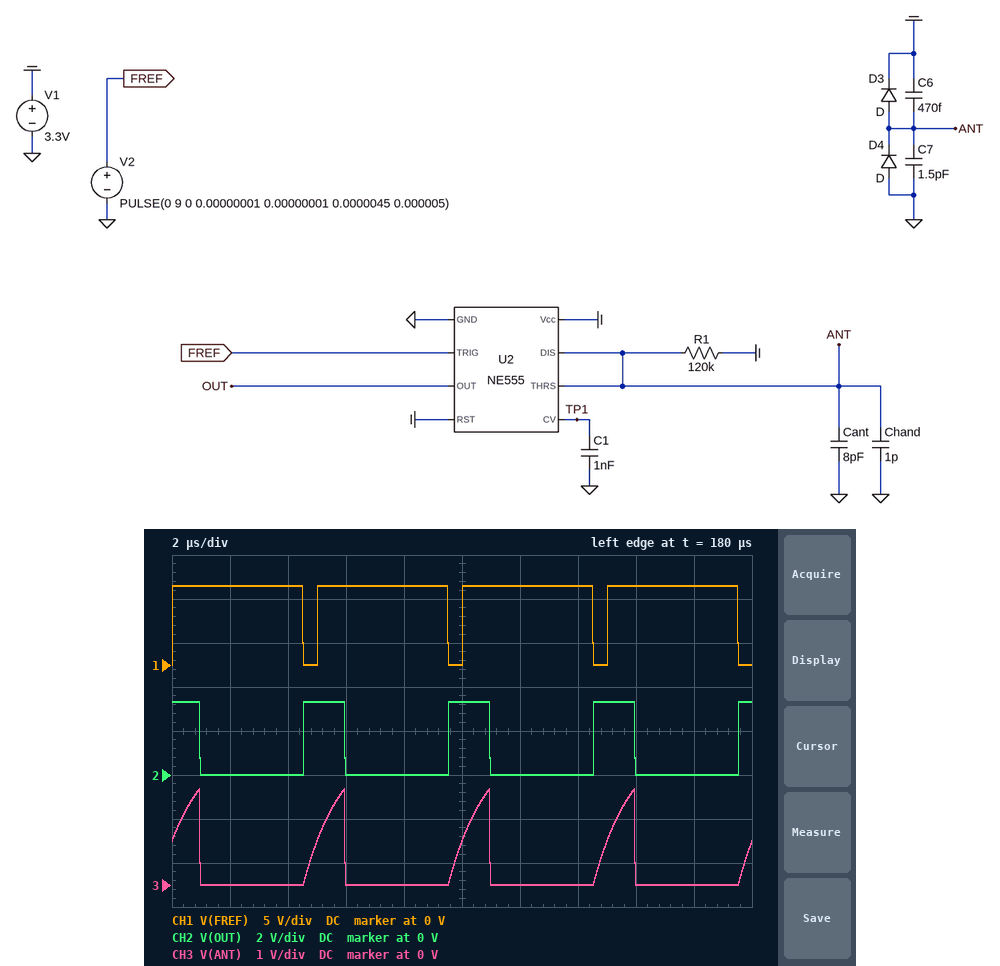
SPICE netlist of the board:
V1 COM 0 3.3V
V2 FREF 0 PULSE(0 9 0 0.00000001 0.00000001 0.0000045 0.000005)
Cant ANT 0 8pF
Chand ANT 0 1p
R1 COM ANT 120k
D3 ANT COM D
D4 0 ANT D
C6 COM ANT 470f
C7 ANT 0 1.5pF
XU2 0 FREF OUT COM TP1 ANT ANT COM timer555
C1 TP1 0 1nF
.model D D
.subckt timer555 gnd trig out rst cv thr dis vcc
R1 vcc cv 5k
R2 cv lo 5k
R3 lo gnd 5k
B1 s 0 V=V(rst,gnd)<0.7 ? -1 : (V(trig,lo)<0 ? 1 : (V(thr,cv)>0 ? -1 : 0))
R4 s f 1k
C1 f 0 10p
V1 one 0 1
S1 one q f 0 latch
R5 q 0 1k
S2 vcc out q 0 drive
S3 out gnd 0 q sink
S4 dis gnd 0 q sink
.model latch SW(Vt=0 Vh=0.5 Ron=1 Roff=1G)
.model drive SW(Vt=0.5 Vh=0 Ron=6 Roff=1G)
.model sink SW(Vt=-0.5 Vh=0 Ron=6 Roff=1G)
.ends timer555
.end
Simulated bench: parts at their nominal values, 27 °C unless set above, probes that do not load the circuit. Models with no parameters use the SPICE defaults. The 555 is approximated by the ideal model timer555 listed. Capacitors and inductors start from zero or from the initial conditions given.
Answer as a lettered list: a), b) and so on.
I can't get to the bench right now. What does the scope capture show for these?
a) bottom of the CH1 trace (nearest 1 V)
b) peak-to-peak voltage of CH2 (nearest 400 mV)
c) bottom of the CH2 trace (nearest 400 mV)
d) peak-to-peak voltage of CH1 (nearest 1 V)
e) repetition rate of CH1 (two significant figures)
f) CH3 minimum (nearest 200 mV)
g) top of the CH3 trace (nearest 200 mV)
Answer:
a) 0 V
b) 3.2 V
c) 0 V
d) 9 V
e) 200 kHz
f) 0 V
g) 2.2 V
